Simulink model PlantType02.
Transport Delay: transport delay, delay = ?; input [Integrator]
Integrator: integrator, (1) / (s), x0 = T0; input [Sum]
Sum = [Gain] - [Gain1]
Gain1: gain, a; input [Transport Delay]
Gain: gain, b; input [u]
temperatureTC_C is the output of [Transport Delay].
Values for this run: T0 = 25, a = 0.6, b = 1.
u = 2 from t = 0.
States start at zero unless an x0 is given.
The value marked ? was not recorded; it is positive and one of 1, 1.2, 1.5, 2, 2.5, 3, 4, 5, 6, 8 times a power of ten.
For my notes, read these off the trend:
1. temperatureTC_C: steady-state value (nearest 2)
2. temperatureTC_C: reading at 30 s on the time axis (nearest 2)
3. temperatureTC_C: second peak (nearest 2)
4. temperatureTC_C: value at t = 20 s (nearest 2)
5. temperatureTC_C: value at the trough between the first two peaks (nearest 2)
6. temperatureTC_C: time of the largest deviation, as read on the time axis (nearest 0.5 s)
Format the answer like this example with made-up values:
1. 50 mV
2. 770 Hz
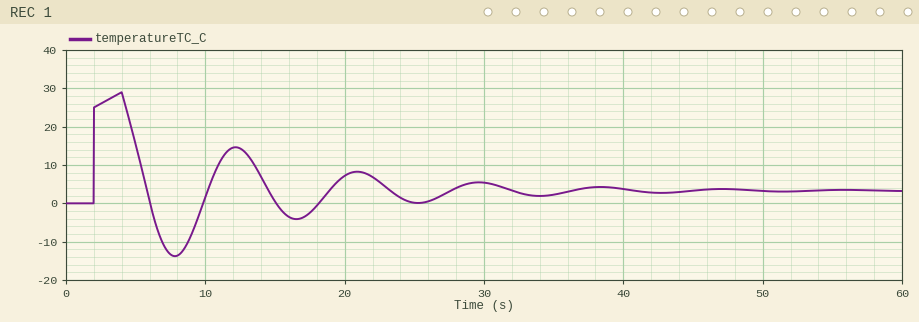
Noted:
1. 4
2. 6
3. 14
4. 8
5. -14
6. 4.0 s
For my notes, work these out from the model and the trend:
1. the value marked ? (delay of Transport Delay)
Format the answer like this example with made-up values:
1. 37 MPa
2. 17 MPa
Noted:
1. 2
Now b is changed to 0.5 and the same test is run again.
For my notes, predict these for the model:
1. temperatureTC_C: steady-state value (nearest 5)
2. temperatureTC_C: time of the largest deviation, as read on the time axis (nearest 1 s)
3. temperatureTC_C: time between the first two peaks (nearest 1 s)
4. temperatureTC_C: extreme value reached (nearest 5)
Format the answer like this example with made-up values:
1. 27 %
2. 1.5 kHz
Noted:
1. 0
2. 4 s
3. 8 s
4. 25
